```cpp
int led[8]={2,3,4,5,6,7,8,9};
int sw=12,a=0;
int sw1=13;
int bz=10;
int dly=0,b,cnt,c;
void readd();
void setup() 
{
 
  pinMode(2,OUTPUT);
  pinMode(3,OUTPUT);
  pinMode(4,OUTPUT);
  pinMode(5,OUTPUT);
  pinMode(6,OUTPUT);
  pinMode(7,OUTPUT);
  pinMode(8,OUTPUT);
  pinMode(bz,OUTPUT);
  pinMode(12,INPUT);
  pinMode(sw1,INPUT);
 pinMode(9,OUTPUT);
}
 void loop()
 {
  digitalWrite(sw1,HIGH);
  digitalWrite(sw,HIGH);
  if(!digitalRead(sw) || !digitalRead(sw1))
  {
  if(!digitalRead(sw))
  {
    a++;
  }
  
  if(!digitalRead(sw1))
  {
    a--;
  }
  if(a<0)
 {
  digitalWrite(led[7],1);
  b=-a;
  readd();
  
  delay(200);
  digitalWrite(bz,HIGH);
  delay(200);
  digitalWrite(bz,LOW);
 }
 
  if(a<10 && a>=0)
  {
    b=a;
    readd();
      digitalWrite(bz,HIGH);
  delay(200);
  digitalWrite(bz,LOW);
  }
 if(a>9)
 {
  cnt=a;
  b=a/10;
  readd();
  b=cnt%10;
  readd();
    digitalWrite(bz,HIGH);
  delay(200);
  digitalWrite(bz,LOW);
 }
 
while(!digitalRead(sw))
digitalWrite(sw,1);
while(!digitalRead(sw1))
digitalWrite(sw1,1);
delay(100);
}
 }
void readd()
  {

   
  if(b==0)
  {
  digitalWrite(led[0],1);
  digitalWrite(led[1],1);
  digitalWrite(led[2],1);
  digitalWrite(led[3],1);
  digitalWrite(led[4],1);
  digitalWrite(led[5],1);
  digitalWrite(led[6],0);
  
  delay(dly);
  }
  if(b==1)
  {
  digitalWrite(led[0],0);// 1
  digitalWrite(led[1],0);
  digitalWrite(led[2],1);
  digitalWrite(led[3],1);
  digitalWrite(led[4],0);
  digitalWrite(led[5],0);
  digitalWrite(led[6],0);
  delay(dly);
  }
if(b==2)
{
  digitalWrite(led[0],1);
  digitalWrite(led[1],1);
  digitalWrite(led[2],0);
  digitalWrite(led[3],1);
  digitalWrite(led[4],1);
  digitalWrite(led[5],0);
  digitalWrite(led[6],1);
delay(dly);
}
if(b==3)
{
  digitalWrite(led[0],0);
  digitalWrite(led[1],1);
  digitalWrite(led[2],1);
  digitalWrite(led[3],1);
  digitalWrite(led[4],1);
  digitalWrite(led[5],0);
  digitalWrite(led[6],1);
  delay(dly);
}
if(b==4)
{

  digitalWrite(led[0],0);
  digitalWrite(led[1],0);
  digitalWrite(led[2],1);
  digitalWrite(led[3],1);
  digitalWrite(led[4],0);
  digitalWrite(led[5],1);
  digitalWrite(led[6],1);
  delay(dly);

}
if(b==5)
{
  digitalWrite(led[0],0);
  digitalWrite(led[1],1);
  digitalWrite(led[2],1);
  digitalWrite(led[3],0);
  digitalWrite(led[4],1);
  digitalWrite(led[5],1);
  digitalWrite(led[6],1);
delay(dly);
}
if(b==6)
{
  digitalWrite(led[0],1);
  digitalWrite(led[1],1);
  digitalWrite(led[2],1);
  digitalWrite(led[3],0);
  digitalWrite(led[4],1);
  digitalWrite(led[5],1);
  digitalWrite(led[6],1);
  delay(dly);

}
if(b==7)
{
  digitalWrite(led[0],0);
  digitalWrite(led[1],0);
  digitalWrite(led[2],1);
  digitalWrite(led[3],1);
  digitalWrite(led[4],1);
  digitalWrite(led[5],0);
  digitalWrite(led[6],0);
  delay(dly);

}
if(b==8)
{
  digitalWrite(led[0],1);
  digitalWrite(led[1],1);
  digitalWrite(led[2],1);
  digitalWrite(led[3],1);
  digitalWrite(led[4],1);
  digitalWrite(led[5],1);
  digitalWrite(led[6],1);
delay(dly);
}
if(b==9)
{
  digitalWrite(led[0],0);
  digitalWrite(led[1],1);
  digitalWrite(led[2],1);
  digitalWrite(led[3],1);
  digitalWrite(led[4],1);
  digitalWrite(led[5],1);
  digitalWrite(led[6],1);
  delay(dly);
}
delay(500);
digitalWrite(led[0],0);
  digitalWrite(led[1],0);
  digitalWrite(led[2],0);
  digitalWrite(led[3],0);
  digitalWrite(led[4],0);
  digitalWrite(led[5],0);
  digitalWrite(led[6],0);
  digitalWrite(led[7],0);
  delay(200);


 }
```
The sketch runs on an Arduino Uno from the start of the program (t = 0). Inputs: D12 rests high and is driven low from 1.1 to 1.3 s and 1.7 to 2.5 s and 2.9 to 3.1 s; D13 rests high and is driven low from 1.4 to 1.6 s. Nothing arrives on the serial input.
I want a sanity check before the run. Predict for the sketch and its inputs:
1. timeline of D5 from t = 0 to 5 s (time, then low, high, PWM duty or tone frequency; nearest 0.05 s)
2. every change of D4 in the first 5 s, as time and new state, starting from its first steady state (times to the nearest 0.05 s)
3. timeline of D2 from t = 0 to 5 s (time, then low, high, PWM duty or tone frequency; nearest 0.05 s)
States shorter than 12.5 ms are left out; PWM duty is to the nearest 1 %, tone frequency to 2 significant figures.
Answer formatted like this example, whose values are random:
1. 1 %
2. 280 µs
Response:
1. 0 s low; 1.1 s high; 1.6 s low; 2.9 s high; 3.4 s low
2. 0 s low; 1.1 s high; 1.6 s low
3. 0 s low; 2.9 s high; 3.4 s low
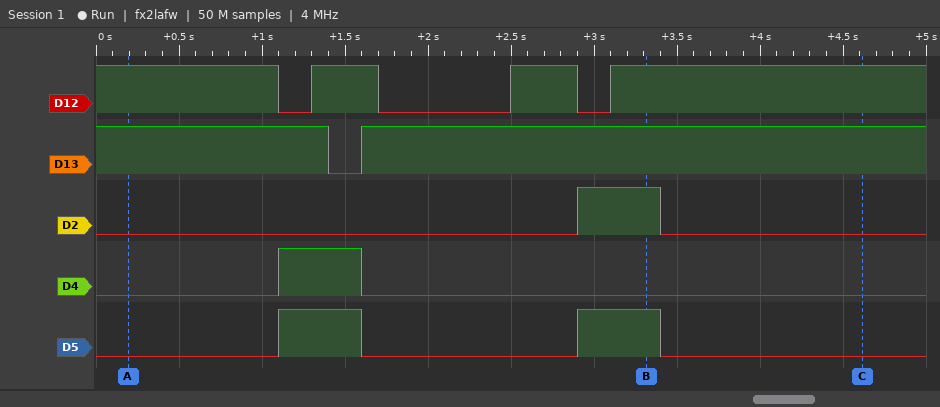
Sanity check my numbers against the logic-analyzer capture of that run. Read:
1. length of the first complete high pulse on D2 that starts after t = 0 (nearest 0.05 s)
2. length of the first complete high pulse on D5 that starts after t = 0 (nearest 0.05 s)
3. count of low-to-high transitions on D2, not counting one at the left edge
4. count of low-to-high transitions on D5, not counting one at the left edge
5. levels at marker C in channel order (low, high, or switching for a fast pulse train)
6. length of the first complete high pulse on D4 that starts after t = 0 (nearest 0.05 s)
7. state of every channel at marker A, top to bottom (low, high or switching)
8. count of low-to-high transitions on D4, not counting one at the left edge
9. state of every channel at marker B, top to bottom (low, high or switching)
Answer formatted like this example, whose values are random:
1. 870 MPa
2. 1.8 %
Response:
1. 0.50 s
2. 0.50 s
3. 1
4. 2
5. D12 high, D13 high, D2 low, D4 low, D5 low
6. 0.50 s
7. D12 high, D13 high, D2 low, D4 low, D5 low
8. 1
9. D12 high, D13 high, D2 high, D4 low, D5 high
